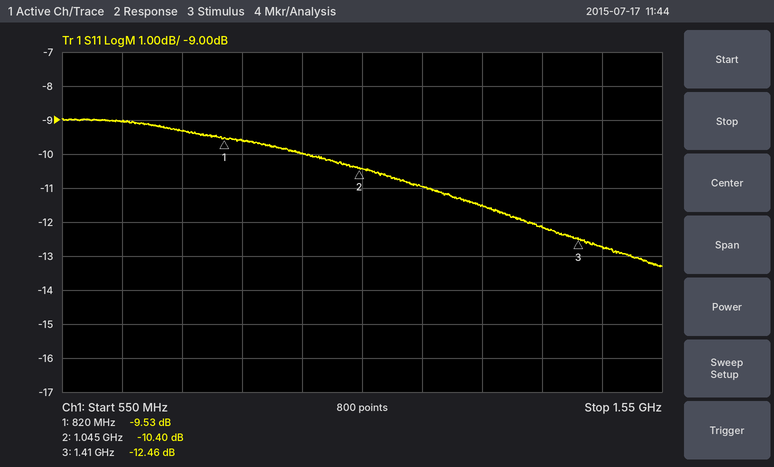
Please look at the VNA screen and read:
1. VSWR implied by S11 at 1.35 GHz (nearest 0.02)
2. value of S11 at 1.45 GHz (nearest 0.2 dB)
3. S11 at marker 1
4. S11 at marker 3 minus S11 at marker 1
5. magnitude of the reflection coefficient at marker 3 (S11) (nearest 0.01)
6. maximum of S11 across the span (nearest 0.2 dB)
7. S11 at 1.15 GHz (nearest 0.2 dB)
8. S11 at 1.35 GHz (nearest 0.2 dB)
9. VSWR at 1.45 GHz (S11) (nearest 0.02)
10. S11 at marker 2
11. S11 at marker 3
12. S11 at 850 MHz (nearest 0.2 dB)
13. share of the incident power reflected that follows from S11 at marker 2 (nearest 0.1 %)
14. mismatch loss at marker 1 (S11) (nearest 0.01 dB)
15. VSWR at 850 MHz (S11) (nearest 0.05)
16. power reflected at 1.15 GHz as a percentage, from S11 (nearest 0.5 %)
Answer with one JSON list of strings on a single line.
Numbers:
["1.66", "-12.8 dB", "-9.53 dB", "-2.93 dB", "0.24", "-9.0 dB", "-11.0 dB", "-12.2 dB", "1.60", "-10.40 dB", "-12.46 dB", "-9.6 dB", "9.1 %", "0.51 dB", "2.00", "8.0 %"]
